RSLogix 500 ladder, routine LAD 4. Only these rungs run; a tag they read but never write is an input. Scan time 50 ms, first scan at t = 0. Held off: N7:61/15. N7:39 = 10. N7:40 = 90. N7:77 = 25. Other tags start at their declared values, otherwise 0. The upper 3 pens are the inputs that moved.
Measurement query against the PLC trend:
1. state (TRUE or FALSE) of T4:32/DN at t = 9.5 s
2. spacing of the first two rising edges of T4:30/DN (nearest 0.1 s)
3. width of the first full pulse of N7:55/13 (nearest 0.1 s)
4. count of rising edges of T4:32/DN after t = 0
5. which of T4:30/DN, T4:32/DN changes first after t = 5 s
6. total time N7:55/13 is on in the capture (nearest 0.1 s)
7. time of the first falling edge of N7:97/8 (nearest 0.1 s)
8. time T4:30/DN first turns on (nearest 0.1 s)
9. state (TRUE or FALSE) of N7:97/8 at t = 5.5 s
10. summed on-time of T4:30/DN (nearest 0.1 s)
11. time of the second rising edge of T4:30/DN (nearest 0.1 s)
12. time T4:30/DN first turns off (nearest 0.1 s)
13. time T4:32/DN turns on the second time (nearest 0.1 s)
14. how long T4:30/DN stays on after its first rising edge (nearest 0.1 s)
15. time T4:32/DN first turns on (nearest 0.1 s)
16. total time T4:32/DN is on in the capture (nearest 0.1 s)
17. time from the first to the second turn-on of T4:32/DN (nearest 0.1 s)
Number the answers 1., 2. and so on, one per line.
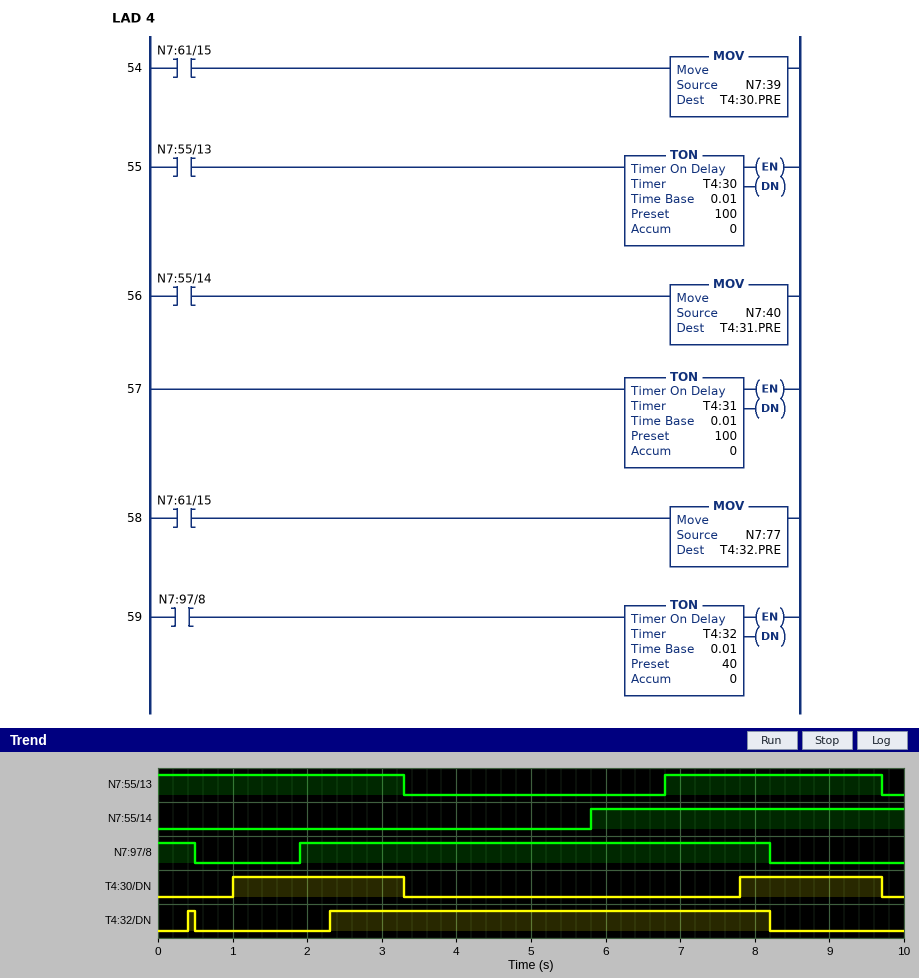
1. FALSE
2. 6.8 s
3. 2.9 s
4. 2
5. T4:30/DN
6. 6.2 s
7. 0.5 s
8. 1.0 s
9. TRUE
10. 4.2 s
11. 7.8 s
12. 3.3 s
13. 2.3 s
14. 2.3 s
15. 0.4 s
16. 6.0 s
17. 1.9 s
